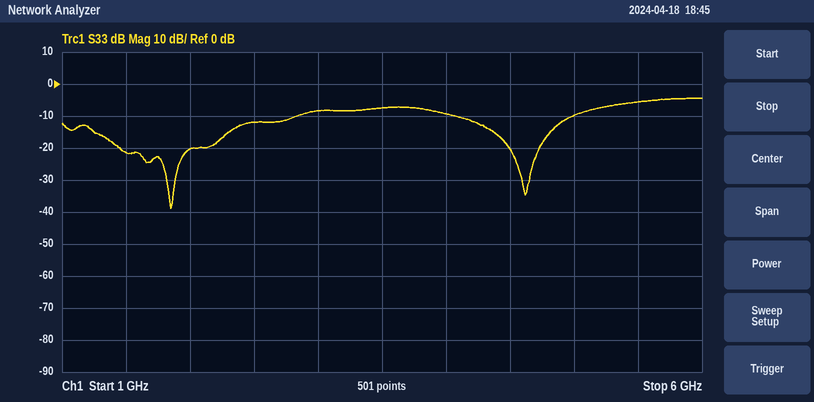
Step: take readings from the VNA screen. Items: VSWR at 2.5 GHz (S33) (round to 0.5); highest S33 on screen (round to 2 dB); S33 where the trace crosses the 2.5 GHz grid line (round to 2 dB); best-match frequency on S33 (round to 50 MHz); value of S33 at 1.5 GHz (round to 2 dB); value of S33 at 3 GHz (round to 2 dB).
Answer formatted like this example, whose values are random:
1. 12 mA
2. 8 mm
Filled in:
1. 1.5
2. -4 dB
3. -12 dB
4. 1.85 GHz
5. -22 dB
6. -8 dB
